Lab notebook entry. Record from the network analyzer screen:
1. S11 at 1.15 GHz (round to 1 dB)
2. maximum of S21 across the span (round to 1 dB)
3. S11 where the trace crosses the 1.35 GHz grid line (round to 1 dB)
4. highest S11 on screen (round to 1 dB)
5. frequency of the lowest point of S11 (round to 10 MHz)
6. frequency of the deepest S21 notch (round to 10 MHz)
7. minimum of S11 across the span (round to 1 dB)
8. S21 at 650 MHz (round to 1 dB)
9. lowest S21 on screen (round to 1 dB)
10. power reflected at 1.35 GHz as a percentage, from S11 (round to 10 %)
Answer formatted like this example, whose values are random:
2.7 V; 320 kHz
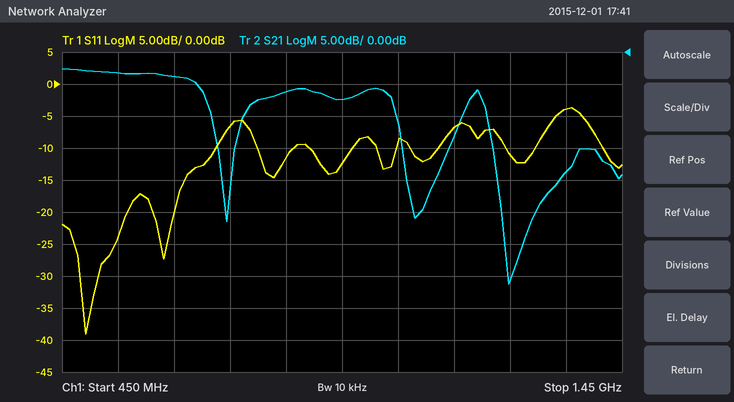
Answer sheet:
-7 dB; -3 dB; -4 dB; -4 dB; 490 MHz; 1.25 GHz; -39 dB; -4 dB; -36 dB; 40 %
